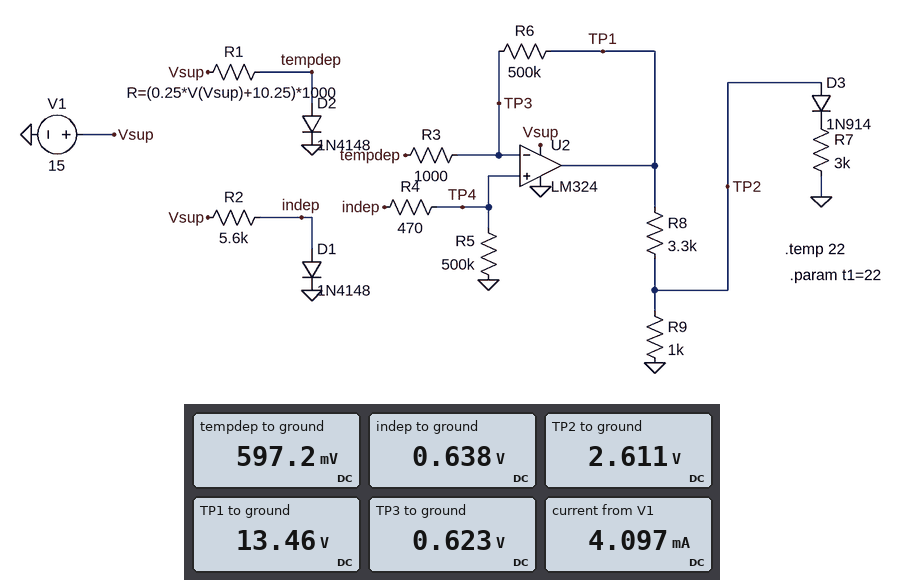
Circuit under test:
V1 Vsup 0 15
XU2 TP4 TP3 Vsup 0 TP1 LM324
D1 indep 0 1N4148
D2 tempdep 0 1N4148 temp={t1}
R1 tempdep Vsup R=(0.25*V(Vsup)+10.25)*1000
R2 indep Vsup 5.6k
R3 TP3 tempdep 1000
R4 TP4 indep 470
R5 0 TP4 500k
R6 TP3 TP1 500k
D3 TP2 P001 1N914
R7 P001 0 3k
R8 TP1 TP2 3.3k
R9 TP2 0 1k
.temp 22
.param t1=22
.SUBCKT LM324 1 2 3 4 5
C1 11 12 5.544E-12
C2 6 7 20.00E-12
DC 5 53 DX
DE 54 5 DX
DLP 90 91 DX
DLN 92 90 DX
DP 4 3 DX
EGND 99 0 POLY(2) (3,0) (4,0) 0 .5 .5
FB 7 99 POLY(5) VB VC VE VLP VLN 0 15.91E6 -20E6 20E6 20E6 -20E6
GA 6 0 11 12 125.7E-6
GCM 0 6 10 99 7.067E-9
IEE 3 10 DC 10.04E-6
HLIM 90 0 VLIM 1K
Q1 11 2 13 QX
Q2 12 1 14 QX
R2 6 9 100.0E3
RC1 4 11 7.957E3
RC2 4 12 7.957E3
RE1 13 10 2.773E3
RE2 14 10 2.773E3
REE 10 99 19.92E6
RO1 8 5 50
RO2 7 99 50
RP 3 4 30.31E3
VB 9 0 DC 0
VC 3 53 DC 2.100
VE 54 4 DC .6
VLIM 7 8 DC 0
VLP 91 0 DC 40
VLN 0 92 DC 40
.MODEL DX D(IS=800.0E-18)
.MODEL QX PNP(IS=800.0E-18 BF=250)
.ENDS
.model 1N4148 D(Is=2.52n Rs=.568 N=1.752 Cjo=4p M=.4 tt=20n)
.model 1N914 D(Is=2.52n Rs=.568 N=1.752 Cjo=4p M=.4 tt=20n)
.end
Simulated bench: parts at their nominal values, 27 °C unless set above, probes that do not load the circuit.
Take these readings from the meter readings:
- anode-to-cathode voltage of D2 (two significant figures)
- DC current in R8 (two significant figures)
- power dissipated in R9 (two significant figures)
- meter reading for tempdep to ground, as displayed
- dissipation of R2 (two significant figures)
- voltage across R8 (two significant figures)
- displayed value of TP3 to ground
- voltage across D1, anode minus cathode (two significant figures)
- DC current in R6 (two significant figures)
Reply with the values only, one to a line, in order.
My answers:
600 mV
3.3 mA
6.8 mW
597.2 mV
37 mW
11 V
0.623 V
640 mV
26 µA
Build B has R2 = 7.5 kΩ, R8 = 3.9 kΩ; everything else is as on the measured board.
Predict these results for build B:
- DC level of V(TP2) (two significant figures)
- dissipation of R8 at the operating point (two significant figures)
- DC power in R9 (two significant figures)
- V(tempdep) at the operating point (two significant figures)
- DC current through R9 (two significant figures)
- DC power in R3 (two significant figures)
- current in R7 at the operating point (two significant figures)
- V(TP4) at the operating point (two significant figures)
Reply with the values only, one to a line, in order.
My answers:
2.3 V
32 mW
5.2 mW
600 mV
2.3 mA
650 nW
570 µA
620 mV
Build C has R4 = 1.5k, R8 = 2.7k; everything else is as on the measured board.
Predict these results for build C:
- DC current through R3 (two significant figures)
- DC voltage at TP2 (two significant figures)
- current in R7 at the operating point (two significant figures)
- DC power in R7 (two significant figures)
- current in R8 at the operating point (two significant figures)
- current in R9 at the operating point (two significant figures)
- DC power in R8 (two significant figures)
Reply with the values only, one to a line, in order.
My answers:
26 µA
3.0 V
820 µA
2.0 mW
3.9 mA
3.0 mA
40 mW
